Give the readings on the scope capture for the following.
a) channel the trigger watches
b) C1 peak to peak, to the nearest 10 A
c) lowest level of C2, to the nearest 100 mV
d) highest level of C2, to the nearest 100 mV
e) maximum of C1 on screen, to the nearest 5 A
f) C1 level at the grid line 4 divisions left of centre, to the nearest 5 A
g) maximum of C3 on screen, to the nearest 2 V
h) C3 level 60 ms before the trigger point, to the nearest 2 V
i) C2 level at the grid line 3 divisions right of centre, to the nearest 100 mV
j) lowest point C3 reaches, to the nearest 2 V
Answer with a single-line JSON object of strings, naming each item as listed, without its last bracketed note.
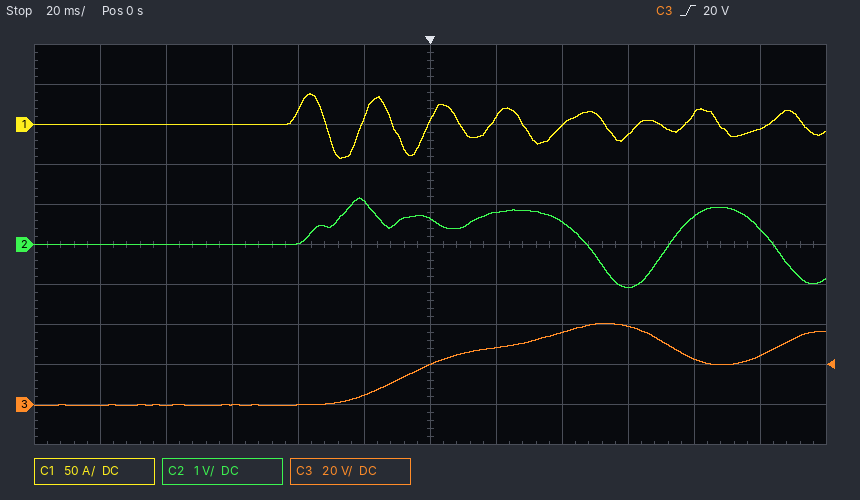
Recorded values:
{"channel the trigger watches": "C3", "C1 peak to peak, to the nearest 10 A": "80 A", "lowest level of C2, to the nearest 100 mV": "-1.1 V", "highest level of C2, to the nearest 100 mV": "1.2 V", "maximum of C1 on screen, to the nearest 5 A": "40 A", "C1 level at the grid line 4 divisions left of centre, to the nearest 5 A": "0 A", "maximum of C3 on screen, to the nearest 2 V": "40 V", "C3 level 60 ms before the trigger point, to the nearest 2 V": "0 V", "C2 level at the grid line 3 divisions right of centre, to the nearest 100 mV": "-1.1 V", "lowest point C3 reaches, to the nearest 2 V": "0 V"}
